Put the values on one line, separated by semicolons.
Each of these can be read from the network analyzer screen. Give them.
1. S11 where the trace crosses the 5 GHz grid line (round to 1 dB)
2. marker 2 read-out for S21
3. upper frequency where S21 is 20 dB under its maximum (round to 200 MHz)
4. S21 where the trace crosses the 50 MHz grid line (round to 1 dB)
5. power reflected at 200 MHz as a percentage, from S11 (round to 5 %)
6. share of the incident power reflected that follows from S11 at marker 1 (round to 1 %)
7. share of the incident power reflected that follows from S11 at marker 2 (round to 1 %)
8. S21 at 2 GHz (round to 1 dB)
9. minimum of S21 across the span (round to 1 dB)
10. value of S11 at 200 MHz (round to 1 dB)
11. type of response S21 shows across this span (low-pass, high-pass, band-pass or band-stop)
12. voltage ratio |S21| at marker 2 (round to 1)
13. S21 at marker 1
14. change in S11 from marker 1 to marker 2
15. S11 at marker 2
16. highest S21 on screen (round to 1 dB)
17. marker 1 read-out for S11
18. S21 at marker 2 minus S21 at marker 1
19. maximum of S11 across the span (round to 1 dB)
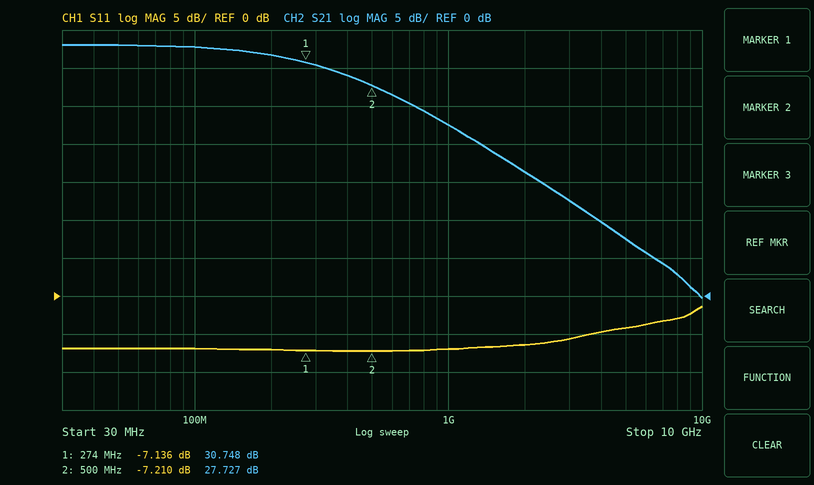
-4 dB; 27.727 dB; 2.8 GHz; 33 dB; 20 %; 19 %; 19 %; 16 dB; 0 dB; -7 dB; low-pass; 24; 30.748 dB; -0.074 dB; -7.210 dB; 33 dB; -7.136 dB; -3.021 dB; -1 dB
